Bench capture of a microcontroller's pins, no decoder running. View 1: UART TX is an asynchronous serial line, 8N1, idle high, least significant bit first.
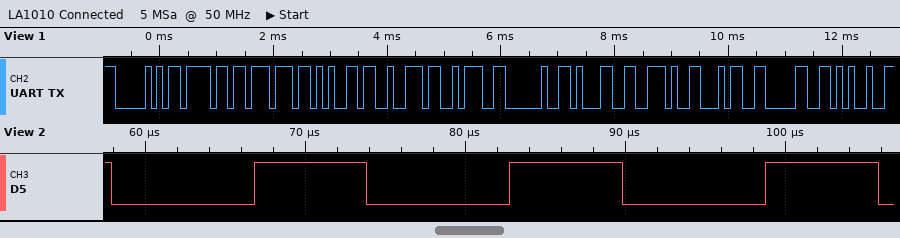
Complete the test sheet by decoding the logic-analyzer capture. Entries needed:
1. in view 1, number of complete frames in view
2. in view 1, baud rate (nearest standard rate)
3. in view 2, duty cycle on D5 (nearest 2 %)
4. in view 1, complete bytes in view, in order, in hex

12
9600 baud
44 %
50 6F 77 65 72 3A 20 31 2E 34 30 25
